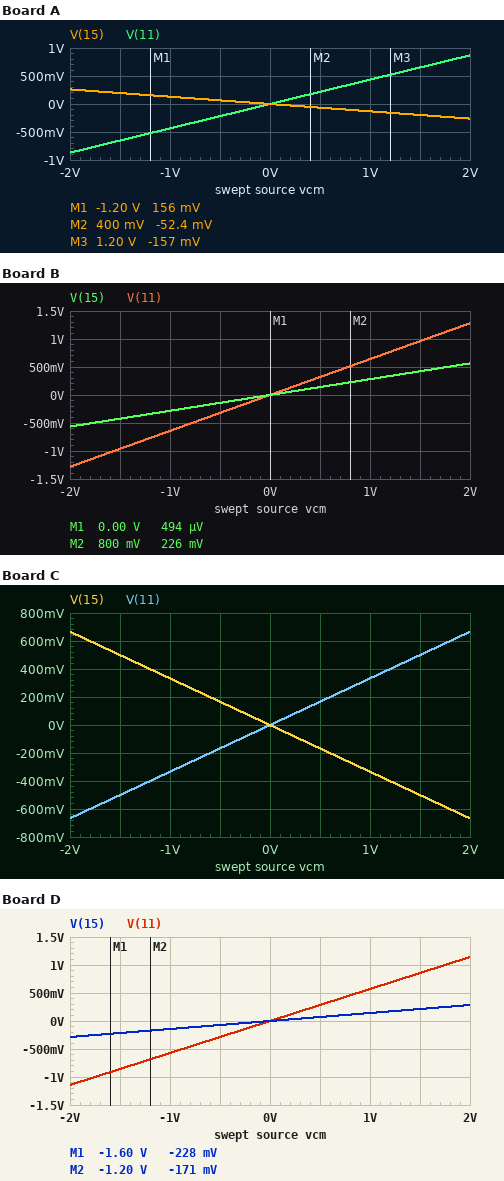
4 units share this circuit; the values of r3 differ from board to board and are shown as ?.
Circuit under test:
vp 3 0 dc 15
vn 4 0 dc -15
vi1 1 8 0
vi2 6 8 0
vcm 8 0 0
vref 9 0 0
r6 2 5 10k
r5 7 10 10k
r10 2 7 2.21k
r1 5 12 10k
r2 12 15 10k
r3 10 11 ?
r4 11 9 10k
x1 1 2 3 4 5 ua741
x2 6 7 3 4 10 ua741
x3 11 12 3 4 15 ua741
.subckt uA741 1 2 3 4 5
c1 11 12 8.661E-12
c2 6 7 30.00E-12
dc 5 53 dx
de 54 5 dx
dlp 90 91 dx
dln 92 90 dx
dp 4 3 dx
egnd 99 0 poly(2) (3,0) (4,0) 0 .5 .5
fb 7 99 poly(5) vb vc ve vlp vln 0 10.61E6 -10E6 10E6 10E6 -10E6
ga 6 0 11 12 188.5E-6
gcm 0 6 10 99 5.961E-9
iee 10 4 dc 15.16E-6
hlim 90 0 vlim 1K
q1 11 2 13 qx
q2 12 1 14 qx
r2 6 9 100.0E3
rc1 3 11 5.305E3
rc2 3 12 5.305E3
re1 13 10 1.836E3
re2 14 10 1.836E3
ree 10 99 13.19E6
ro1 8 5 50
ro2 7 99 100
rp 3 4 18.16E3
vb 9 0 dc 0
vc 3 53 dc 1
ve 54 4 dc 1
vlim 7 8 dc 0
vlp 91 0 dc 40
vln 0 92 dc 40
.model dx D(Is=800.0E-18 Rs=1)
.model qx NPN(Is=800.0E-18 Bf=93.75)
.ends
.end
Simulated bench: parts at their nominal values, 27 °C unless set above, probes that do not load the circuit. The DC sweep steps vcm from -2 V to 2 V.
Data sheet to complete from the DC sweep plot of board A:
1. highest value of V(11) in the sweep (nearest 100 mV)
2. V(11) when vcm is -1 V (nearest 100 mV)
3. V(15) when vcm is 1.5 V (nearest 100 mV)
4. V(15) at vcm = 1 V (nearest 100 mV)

900 mV
-400 mV
-200 mV
-100 mV
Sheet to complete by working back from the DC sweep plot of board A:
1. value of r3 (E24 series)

13 kΩ
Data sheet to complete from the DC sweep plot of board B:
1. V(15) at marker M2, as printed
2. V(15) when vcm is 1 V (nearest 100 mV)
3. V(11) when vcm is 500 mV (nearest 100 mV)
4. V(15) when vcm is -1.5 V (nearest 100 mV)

226 mV
300 mV
300 mV
-400 mV
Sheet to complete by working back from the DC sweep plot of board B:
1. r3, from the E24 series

5.6 kΩ
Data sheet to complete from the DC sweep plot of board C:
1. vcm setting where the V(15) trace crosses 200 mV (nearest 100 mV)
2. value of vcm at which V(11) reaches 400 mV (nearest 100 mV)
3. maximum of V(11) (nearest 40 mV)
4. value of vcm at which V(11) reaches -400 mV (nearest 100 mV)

-600 mV
1.2 V
680 mV
-1.2 V
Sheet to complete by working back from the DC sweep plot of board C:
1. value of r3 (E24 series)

20 kΩ
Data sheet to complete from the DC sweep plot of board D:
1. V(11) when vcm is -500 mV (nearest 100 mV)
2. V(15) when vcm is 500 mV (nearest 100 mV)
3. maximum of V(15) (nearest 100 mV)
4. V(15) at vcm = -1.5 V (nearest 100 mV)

-300 mV
100 mV
300 mV
-200 mV
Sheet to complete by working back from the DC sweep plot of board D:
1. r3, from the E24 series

7.5 kΩ
